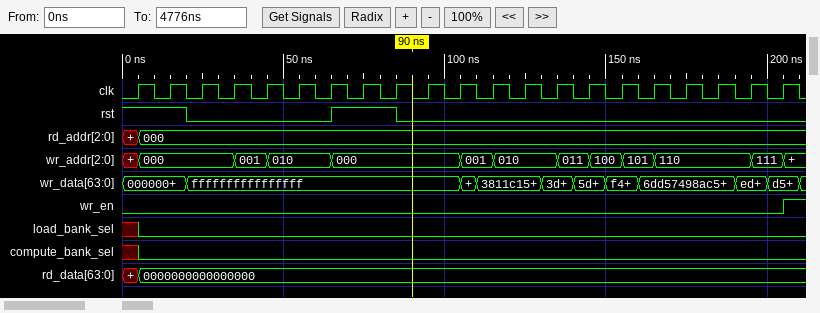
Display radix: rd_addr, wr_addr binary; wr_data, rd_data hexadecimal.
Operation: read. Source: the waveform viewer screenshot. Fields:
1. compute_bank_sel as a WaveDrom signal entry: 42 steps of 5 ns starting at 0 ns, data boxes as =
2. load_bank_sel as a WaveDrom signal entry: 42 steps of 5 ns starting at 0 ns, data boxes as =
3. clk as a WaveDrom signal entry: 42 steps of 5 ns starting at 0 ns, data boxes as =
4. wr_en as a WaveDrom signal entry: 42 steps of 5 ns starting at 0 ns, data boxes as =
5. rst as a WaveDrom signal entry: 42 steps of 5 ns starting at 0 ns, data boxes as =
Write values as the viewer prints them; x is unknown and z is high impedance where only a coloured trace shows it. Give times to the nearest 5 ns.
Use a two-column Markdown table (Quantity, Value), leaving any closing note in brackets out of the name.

| Quantity | Value |
|---|---|
| compute_bank_sel as a WaveDrom signal entry: 42 steps of 5 ns starting at 0 ns, data boxes as = | {name: 'compute_bank_sel', wave: 'x0........................................'} |
| load_bank_sel as a WaveDrom signal entry: 42 steps of 5 ns starting at 0 ns, data boxes as = | {name: 'load_bank_sel', wave: 'x0........................................'} |
| clk as a WaveDrom signal entry: 42 steps of 5 ns starting at 0 ns, data boxes as = | {name: 'clk', wave: '010101010101010101010101010101010101010101'} |
| wr_en as a WaveDrom signal entry: 42 steps of 5 ns starting at 0 ns, data boxes as = | {name: 'wr_en', wave: '0........................................1'} |
| rst as a WaveDrom signal entry: 42 steps of 5 ns starting at 0 ns, data boxes as = | {name: 'rst', wave: '1...0........1...0........................'} |
